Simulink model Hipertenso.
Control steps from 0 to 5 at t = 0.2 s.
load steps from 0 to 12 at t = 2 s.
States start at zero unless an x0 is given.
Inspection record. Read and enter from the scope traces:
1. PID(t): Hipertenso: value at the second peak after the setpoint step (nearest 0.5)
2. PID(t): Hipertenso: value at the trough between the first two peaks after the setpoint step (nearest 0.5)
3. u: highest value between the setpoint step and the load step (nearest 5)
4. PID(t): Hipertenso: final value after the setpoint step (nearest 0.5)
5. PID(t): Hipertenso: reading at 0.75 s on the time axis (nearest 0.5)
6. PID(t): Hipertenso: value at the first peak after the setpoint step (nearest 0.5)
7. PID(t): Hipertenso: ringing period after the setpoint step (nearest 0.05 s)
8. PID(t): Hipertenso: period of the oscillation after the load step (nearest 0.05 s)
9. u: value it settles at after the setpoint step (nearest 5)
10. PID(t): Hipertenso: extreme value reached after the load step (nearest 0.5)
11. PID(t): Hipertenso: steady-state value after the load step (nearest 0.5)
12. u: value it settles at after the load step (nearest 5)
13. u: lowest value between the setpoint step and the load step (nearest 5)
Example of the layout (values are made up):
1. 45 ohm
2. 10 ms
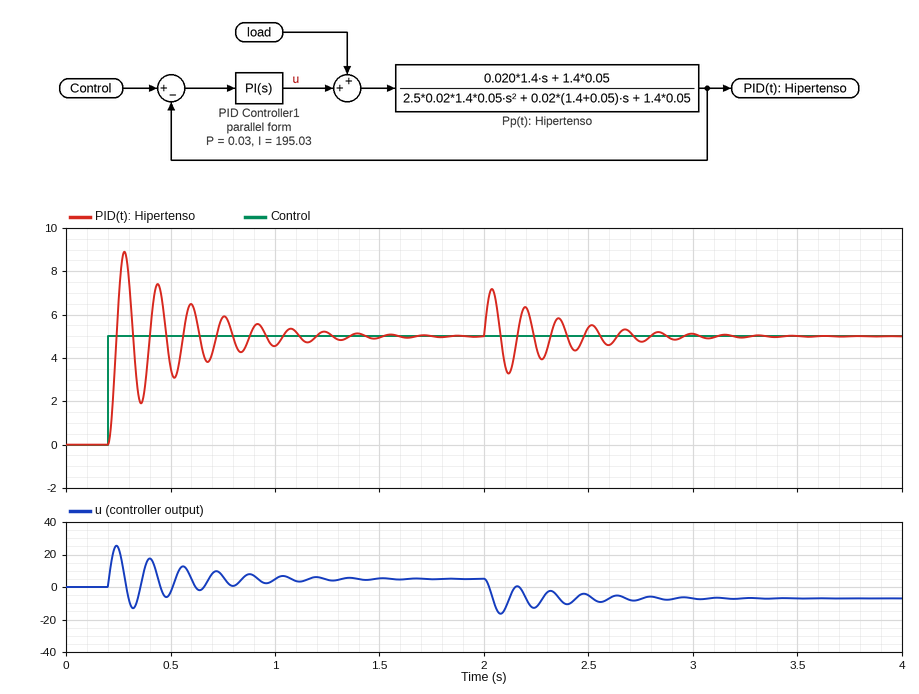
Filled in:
1. 7.5
2. 2.0
3. 25
4. 5.0
5. 6.0
6. 9.0
7. 0.15 s
8. 0.15 s
9. 5
10. 7.0
11. 5.0
12. -5
13. -15
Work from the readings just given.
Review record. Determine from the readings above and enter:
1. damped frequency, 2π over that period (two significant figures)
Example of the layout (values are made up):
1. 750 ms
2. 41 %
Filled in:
1. 42 rad/s
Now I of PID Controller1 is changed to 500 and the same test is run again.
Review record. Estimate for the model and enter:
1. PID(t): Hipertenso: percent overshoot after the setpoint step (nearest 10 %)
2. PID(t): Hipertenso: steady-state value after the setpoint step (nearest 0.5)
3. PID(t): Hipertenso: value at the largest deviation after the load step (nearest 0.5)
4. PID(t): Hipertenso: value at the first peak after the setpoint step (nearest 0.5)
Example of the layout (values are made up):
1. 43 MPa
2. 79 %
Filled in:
1. 90 %
2. 5.0
3. 6.5
4. 9.5
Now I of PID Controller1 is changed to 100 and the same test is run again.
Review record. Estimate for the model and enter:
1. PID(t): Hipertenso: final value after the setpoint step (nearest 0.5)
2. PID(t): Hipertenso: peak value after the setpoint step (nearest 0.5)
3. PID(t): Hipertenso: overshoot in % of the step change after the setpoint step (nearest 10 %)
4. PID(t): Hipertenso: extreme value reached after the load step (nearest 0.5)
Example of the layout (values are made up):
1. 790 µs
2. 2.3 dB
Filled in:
1. 5.0
2. 8.5
3. 70 %
4. 8.0
